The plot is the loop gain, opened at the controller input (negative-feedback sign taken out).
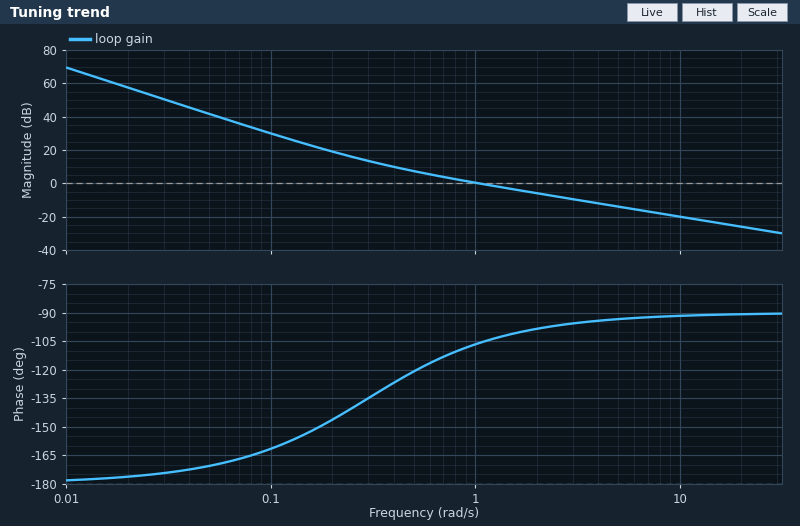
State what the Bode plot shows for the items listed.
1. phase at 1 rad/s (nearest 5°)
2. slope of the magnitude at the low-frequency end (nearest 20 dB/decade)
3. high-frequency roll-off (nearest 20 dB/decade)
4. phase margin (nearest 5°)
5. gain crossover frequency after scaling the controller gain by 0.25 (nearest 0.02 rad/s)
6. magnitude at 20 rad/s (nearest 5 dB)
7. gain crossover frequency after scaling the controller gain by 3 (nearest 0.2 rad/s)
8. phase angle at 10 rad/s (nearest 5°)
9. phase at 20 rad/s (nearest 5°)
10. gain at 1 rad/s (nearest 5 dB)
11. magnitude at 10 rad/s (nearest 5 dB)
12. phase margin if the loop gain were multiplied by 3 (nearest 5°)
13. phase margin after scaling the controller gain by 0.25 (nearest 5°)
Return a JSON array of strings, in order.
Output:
["-105°", "-40 dB/decade", "-20 dB/decade", "75°", "0.34 rad/s", "-25 dB", "3.0 rad/s", "-90°", "-90°", "0 dB", "-20 dB", "85°", "50°"]
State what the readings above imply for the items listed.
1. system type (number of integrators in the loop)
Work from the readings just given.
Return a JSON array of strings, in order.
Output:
["2"]
